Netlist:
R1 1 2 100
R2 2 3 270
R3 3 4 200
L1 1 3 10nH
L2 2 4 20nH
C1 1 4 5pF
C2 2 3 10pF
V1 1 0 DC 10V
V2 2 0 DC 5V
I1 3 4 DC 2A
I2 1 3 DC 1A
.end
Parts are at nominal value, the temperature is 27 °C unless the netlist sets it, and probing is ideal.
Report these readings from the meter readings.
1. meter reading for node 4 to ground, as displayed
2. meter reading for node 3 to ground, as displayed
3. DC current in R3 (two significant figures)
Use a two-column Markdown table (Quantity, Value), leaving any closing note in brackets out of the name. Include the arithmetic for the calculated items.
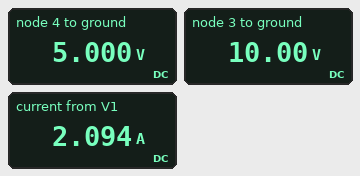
| Quantity | Value |
|---|---|
| meter reading for node 4 to ground, as displayed | 5.000 V |
| meter reading for node 3 to ground, as displayed | 10.00 V |
| DC current in R3 | (10 V - 5 V) / 200 Ω = 25 mA |
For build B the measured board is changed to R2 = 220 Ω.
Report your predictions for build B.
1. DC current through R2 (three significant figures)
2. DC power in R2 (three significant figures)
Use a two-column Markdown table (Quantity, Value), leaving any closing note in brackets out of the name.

| Quantity | Value |
|---|---|
| DC current through R2 | 22.7 mA |
| DC power in R2 | 114 mW |
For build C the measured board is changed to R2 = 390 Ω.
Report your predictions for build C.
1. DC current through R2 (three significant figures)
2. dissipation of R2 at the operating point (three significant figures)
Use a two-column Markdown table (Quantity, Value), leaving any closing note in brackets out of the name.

| Quantity | Value |
|---|---|
| DC current through R2 | 12.8 mA |
| dissipation of R2 at the operating point | 64.1 mW |
